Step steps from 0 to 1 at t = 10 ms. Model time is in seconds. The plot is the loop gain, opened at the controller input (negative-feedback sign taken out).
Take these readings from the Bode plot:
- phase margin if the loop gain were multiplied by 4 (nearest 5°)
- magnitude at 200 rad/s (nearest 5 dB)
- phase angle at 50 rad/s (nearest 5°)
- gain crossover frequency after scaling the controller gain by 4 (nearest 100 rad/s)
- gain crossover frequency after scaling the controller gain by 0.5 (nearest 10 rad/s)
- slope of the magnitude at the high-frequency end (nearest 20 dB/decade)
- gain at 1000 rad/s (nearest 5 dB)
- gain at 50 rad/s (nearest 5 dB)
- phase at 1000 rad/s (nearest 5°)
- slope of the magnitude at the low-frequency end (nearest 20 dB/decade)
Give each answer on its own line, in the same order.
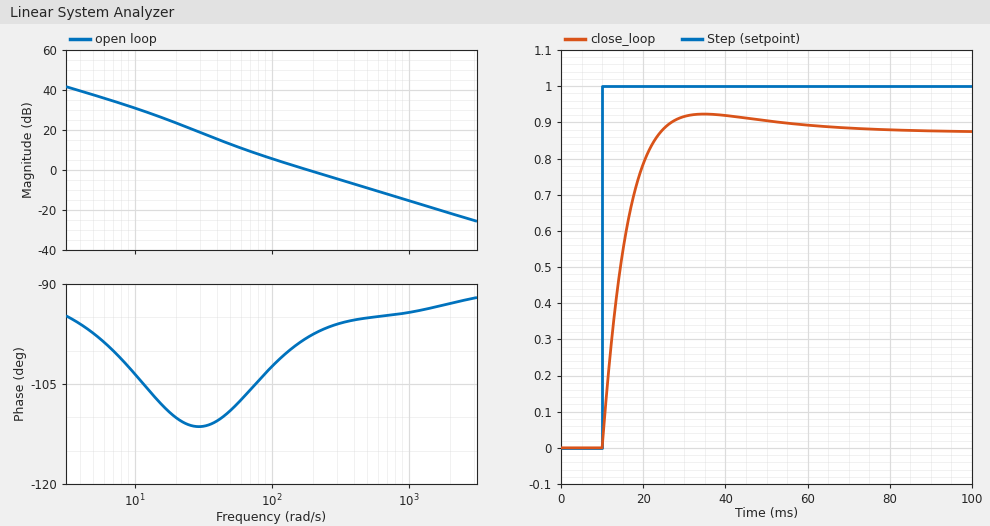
85°
0 dB
-110°
700 rad/s
100 rad/s
-20 dB/decade
-15 dB
15 dB
-95°
-20 dB/decade
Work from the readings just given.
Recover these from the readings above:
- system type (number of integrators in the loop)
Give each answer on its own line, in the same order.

1
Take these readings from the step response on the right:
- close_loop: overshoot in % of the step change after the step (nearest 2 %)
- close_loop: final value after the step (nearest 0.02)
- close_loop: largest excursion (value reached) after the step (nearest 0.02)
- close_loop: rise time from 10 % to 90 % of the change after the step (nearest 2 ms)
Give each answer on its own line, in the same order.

6 %
0.88
0.92
10 ms
